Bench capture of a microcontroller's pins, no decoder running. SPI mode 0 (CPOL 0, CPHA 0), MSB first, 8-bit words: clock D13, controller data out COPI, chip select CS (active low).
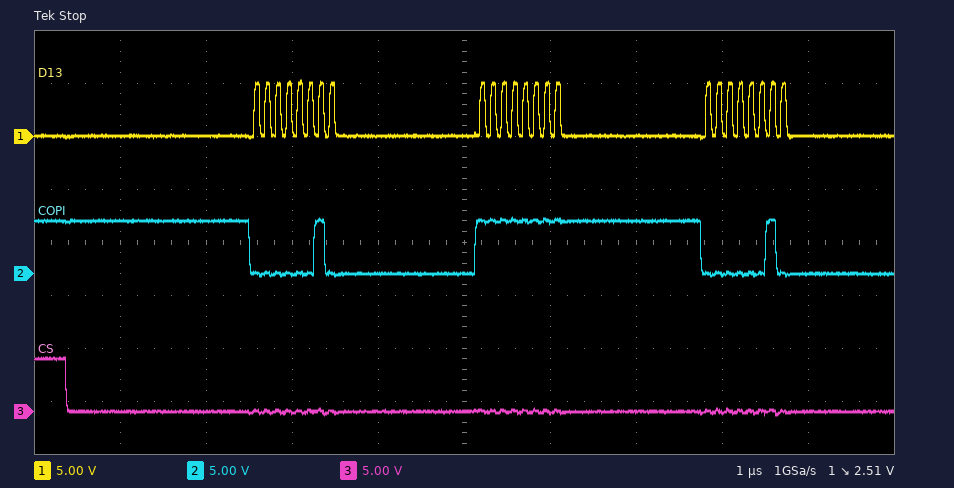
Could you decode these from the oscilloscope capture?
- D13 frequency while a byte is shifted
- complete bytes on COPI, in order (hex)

8 MHz
0x02 0xFF 0x02
